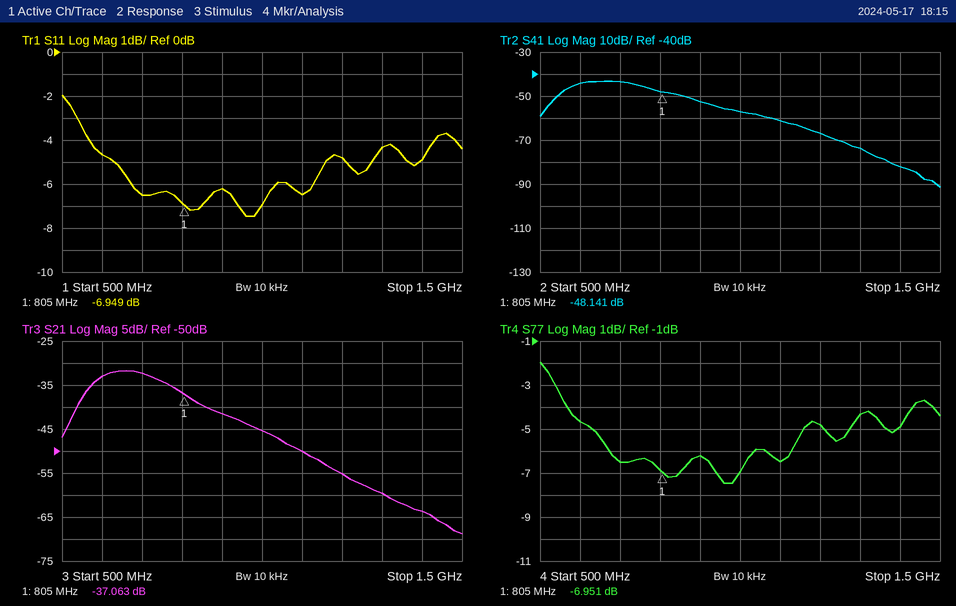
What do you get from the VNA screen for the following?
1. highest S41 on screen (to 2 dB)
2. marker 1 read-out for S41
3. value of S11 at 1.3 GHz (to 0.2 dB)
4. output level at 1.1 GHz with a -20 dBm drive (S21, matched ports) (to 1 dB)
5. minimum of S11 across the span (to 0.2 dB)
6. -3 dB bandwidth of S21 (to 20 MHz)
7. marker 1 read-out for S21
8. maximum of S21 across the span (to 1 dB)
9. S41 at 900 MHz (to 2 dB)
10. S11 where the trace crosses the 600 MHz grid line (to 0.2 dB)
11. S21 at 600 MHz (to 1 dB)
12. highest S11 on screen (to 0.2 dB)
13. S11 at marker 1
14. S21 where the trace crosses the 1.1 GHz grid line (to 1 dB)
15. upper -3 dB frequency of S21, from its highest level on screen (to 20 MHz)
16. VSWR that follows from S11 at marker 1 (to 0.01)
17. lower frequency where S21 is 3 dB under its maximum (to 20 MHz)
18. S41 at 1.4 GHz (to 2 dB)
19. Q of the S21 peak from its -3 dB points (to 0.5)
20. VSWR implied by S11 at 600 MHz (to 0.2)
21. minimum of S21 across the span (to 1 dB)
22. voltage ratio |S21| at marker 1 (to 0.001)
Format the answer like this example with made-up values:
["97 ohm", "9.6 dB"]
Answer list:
["-44 dB", "-48.141 dB", "-4.4 dB", "-70 dBm", "-7.4 dB", "180 MHz", "-37.063 dB", "-32 dB", "-52 dB", "-4.6 dB", "-33 dB", "-2.0 dB", "-6.949 dB", "-50 dB", "760 MHz", "2.63", "580 MHz", "-82 dB", "3.5", "3.8", "-69 dB", "0.014"]
